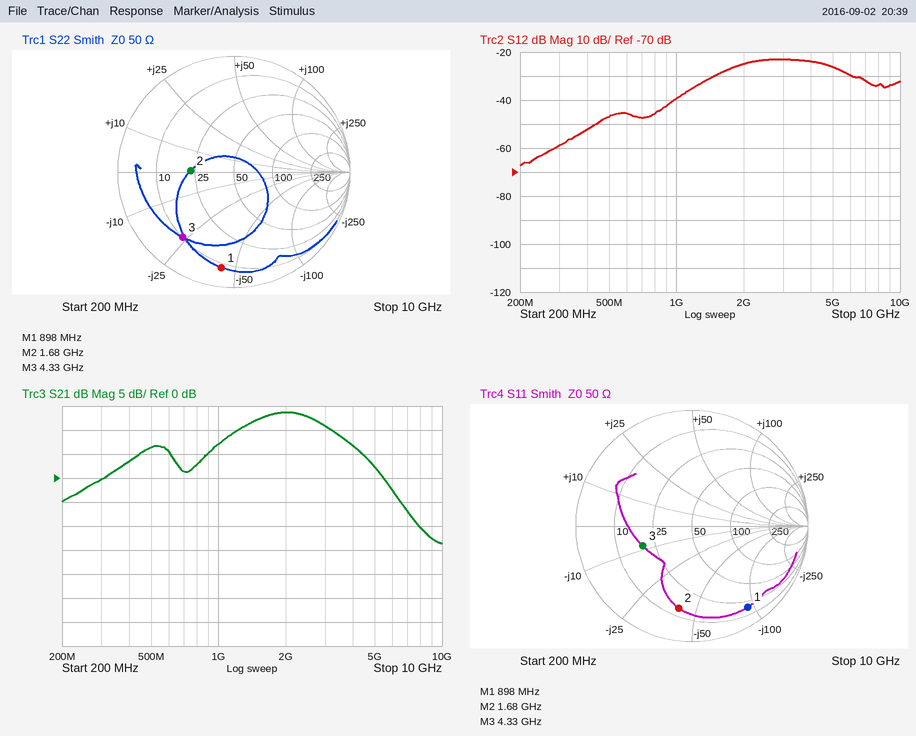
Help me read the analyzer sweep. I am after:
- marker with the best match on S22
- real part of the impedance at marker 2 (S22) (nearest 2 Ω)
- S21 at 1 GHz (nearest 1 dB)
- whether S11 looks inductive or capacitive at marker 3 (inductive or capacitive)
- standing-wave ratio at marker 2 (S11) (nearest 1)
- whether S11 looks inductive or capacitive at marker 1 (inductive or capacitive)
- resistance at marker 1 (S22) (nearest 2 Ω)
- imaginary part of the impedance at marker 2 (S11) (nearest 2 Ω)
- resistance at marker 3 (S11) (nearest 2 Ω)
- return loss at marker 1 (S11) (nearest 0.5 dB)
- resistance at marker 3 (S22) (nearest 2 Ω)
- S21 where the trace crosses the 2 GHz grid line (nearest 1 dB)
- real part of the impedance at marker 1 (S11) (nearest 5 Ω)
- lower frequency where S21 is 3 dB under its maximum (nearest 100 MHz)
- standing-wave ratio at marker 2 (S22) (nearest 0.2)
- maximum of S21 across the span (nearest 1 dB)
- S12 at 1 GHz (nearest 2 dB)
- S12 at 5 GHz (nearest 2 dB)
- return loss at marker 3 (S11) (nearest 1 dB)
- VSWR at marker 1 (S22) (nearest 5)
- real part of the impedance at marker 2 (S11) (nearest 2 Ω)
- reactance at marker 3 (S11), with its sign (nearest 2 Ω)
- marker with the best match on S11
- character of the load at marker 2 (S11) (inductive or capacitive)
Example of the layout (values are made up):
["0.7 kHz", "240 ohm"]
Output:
["marker 2", "22 Ω", "7 dB", "capacitive", "6", "capacitive", "8 Ω", "-40 Ω", "20 Ω", "1.5 dB", "10 Ω", "14 dB", "20 Ω", "1.3 GHz", "2.2", "14 dB", "-40 dB", "-26 dB", "7 dB", "10", "14 Ω", "-8 Ω", "marker 3", "capacitive"]
